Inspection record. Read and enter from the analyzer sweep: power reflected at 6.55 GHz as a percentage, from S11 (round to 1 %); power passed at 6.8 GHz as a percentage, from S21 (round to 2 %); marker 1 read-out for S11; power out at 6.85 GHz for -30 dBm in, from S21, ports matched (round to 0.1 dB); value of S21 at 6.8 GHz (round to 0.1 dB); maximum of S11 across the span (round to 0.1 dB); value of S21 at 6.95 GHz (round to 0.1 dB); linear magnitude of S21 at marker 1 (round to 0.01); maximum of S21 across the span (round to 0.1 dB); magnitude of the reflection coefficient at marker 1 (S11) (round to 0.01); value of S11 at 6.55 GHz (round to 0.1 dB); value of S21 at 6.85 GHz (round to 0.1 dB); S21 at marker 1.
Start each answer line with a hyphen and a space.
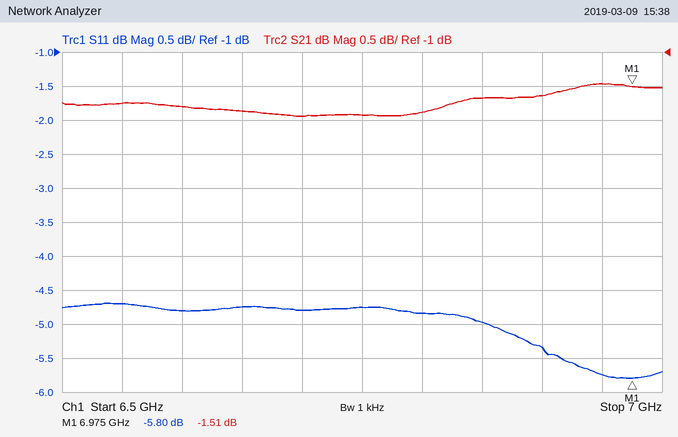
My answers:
- 34 %
- 64 %
- -5.80 dB
- -31.7 dBm
- -1.9 dB
- -4.7 dB
- -1.5 dB
- 0.84
- -1.5 dB
- 0.51
- -4.7 dB
- -1.7 dB
- -1.51 dB
